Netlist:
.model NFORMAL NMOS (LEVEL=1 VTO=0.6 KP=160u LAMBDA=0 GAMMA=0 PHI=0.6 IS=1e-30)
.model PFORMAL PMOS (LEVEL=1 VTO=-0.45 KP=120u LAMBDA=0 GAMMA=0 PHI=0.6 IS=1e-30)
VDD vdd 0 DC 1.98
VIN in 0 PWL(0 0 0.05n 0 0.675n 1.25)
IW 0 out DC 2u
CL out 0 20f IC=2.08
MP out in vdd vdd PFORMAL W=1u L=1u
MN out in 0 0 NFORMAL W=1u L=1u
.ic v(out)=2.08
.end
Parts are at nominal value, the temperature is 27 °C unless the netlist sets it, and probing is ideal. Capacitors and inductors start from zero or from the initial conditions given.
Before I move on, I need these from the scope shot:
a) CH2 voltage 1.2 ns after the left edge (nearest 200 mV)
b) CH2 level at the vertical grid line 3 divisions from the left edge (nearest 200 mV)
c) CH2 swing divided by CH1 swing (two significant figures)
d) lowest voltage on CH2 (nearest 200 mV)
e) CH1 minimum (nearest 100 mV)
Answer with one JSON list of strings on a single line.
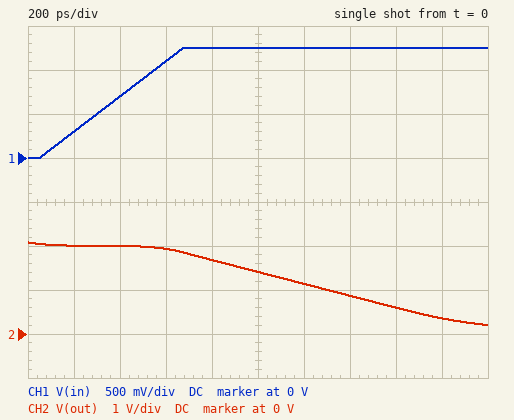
["1.2 V", "2.0 V", "1.5", "200 mV", "0 V"]
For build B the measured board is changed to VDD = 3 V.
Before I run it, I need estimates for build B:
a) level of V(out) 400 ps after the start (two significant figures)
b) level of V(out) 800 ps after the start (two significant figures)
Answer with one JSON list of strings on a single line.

["3.0 V", "2.8 V"]
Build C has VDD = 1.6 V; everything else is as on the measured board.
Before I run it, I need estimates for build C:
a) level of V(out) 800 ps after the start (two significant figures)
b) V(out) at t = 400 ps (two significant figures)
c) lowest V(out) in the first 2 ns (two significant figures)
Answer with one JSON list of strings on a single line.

["1.3 V", "1.7 V", "42 mV"]
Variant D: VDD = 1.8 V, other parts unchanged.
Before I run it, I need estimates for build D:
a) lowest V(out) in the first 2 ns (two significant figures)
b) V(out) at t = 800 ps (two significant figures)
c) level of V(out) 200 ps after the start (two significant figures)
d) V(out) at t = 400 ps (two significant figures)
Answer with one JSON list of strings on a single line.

["68 mV", "1.5 V", "1.9 V", "1.8 V"]
